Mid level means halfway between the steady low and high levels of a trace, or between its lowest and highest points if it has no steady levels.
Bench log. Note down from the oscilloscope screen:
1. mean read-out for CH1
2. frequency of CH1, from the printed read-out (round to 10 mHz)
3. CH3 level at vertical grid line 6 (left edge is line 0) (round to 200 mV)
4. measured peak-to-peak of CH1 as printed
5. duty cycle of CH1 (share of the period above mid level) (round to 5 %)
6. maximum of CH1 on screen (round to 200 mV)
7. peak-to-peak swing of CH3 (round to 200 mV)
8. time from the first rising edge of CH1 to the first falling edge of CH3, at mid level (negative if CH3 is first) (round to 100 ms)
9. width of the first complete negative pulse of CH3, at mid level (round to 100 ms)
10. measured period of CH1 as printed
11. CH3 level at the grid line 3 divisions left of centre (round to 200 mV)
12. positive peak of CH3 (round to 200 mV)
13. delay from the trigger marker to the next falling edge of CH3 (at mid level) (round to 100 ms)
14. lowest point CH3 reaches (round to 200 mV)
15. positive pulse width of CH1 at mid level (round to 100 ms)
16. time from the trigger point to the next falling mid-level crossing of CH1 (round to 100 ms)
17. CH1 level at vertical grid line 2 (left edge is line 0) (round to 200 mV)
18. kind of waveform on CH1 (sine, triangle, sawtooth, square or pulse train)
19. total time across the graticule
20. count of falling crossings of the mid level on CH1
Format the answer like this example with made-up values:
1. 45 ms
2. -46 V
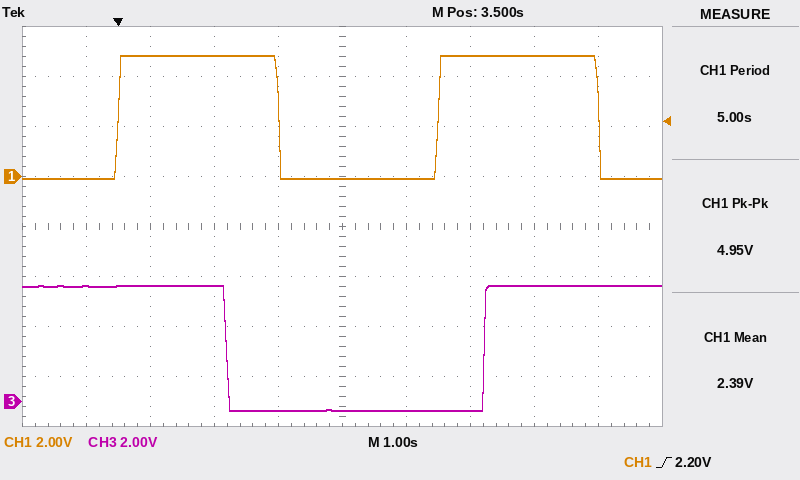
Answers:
1. 2.39 V
2. 200 mHz
3. -400 mV
4. 4.95 V
5. 50 %
6. 4.8 V
7. 5.0 V
8. +1.7 s
9. 4.0 s
10. 5.00 s
11. 4.6 V
12. 4.6 V
13. 1.7 s
14. -400 mV
15. 2.5 s
16. 2.5 s
17. 4.8 V
18. square
19. 10 s
20. 2
